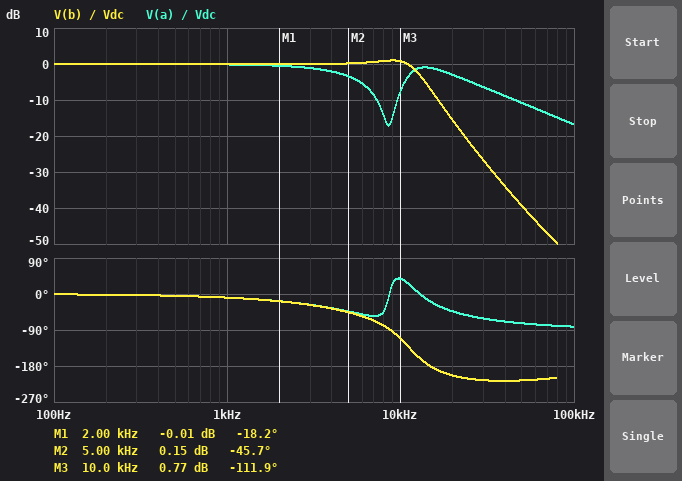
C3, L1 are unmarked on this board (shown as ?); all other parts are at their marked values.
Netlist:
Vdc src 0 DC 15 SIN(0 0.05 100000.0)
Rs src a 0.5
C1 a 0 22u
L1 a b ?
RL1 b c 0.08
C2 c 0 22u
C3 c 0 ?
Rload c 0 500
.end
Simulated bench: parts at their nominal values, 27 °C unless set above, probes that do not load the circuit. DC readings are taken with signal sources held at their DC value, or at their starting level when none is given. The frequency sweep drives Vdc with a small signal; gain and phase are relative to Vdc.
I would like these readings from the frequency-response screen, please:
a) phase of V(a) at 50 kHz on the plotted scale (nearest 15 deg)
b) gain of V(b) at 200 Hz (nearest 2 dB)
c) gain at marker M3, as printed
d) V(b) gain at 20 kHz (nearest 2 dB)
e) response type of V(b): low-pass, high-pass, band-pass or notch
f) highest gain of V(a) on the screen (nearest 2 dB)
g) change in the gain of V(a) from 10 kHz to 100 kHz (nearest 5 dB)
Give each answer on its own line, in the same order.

-75 deg
0 dB
0.77 dB
-16 dB
low-pass
0 dB
-10 dB
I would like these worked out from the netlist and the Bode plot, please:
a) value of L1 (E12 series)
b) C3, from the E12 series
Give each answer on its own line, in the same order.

12 µH
6.8 µF
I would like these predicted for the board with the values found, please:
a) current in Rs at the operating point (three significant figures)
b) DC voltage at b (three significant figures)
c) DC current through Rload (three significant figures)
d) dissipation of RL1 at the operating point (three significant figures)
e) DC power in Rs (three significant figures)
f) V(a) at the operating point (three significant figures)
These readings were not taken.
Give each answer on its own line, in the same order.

30.0 mA
15.0 V
30.0 mA
71.8 µW
449 µW
15.0 V
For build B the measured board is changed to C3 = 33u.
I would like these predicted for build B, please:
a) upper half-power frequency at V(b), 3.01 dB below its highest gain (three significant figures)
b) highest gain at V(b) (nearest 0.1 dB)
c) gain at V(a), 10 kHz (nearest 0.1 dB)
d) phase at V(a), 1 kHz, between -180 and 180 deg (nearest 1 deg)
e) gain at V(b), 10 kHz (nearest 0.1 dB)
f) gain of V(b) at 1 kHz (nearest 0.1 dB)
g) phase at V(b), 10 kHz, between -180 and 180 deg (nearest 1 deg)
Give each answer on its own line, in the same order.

7.90 kHz
0 dB
-1.8 dB
-14 deg
-5.7 dB
-0.1 dB
-138 deg
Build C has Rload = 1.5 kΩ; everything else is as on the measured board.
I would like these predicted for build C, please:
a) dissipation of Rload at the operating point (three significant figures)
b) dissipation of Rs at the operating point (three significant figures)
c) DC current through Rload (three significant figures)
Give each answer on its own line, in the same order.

150 mW
50.0 µW
10.0 mA
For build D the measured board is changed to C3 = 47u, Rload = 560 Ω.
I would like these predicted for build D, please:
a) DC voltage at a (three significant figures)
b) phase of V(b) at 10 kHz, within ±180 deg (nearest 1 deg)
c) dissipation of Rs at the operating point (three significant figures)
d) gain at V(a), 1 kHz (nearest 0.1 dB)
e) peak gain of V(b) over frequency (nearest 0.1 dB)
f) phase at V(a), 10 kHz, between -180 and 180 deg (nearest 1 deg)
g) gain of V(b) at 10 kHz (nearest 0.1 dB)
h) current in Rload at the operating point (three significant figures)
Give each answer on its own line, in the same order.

15.0 V
-140 deg
358 µW
-0.4 dB
0 dB
12 deg
-8.1 dB
26.8 mA
